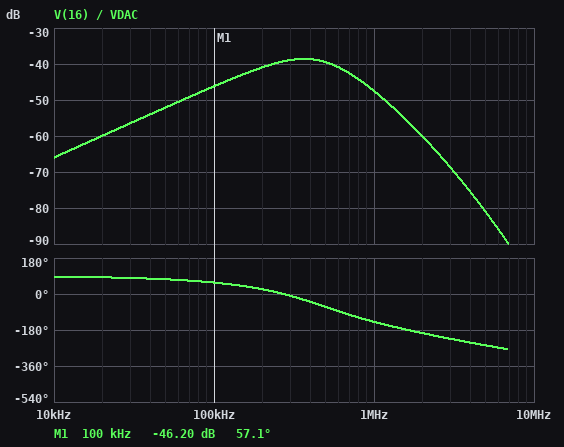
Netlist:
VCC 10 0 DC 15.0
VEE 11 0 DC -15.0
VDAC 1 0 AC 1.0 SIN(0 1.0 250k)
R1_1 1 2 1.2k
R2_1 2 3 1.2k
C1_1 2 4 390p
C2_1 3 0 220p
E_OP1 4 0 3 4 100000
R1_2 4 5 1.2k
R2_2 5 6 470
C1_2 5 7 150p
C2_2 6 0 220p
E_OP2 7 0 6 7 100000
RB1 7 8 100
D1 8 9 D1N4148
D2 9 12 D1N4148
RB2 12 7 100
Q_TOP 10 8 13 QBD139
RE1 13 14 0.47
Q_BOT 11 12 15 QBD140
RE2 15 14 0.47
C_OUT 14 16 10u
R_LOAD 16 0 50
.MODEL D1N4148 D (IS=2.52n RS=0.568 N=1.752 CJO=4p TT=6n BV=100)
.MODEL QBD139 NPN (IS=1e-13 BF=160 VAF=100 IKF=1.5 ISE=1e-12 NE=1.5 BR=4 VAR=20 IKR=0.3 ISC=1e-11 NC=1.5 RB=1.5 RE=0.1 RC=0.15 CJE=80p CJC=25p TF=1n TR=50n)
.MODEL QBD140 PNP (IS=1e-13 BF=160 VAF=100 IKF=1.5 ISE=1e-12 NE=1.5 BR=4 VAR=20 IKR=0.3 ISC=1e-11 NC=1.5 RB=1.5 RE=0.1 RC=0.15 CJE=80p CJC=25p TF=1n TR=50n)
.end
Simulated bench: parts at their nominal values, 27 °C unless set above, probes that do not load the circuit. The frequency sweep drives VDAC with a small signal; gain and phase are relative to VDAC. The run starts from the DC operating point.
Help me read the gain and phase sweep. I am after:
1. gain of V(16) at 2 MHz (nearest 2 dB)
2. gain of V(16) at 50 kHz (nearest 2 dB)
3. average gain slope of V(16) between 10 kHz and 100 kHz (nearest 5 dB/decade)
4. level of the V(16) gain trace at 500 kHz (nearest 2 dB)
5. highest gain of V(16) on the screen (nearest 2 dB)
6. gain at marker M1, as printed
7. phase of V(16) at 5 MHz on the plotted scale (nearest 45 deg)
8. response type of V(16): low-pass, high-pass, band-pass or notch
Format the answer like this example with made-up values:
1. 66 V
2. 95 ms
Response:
1. -60 dB
2. -52 dB
3. 20 dB/decade
4. -40 dB
5. -38 dB
6. -46.20 dB
7. -270 deg
8. band-pass
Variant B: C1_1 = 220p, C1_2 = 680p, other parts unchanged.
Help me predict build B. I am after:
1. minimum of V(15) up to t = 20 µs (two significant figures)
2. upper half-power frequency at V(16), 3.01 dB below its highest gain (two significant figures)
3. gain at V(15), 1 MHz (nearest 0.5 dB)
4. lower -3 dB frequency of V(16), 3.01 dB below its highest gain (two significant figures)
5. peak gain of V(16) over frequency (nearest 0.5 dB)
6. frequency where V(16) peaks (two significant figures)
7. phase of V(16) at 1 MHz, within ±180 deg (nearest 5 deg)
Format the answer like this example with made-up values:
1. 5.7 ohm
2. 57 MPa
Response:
1. -230 mV
2. 660 kHz
3. -48.0 dB
4. 210 kHz
5. -37.5 dB
6. 410 kHz
7. -170 deg
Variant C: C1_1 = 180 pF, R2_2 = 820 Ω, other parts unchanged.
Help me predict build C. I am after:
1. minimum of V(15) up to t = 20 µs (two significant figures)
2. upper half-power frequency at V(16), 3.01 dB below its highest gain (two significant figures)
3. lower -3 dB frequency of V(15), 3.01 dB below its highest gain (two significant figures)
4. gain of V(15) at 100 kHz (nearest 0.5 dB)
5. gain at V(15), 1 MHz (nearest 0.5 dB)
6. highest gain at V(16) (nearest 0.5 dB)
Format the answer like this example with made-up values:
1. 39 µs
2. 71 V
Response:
1. -110 mV
2. 760 kHz
3. 160 kHz
4. -46.5 dB
5. -46.0 dB
6. -40.0 dB
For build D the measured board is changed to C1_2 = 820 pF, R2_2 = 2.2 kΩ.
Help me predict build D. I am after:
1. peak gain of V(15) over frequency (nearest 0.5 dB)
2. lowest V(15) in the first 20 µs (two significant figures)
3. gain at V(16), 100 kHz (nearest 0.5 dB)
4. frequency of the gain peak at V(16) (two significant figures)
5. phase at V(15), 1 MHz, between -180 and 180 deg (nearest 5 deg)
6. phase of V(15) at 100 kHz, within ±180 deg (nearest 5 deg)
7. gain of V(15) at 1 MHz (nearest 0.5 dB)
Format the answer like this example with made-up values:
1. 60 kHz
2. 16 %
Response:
1. -40.0 dB
2. -170 mV
3. -45.5 dB
4. 220 kHz
5. 140 deg
6. 40 deg
7. -65.5 dB
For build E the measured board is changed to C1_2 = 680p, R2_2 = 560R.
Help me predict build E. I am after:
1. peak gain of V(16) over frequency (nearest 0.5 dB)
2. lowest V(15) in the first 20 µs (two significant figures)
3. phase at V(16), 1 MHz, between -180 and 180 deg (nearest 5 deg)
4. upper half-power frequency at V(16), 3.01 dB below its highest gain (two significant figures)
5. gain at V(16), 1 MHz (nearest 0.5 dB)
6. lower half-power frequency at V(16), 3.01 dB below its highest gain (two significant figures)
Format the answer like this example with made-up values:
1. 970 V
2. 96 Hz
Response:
1. -37.0 dB
2. -310 mV
3. 165 deg
4. 570 kHz
5. -52.0 dB
6. 210 kHz
